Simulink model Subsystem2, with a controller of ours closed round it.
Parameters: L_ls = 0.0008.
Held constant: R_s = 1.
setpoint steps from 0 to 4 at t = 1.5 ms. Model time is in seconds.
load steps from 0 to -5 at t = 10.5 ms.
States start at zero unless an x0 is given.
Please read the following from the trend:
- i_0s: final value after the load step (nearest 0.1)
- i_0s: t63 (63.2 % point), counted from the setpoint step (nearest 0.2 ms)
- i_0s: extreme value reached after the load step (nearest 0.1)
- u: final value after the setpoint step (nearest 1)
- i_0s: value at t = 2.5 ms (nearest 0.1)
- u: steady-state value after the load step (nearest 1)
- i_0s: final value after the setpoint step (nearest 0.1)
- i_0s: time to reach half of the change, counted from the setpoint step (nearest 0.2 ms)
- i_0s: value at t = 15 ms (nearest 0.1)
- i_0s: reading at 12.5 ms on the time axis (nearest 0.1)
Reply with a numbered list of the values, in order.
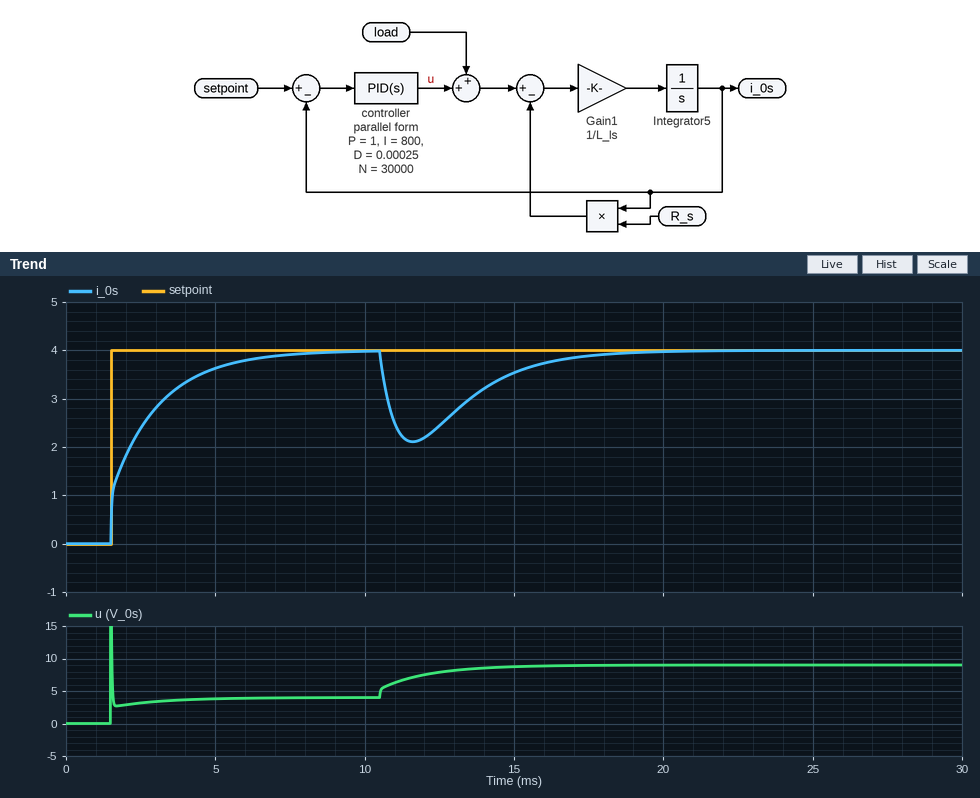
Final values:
1. 4.0
2. 1.2 ms
3. 2.1
4. 4
5. 2.4
6. 9
7. 4.0
8. 0.6 ms
9. 3.5
10. 2.4
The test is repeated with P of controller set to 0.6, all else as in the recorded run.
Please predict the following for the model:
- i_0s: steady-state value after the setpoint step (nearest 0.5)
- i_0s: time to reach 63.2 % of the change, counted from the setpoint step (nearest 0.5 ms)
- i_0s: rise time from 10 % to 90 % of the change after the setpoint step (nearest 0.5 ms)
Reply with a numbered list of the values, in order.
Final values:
1. 4.0
2. 1.5 ms
3. 3.0 ms
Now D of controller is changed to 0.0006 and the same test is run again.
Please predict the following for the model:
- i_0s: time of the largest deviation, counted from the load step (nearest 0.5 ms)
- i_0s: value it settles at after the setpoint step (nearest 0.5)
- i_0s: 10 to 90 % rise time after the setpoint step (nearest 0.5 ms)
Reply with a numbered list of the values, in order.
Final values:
1. 1.5 ms
2. 4.0
3. 3.5 ms
